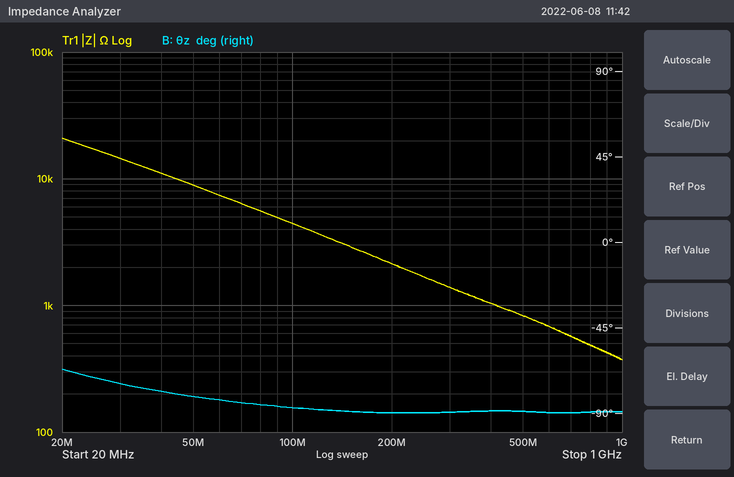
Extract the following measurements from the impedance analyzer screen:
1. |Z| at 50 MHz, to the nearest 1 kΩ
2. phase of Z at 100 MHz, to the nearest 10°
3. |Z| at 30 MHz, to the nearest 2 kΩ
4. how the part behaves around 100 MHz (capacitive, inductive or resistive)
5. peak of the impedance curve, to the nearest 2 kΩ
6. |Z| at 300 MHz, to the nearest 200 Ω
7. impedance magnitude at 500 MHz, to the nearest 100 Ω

9 kΩ
-90°
14 kΩ
capacitive
20 kΩ
1.4 kΩ
800 Ω
